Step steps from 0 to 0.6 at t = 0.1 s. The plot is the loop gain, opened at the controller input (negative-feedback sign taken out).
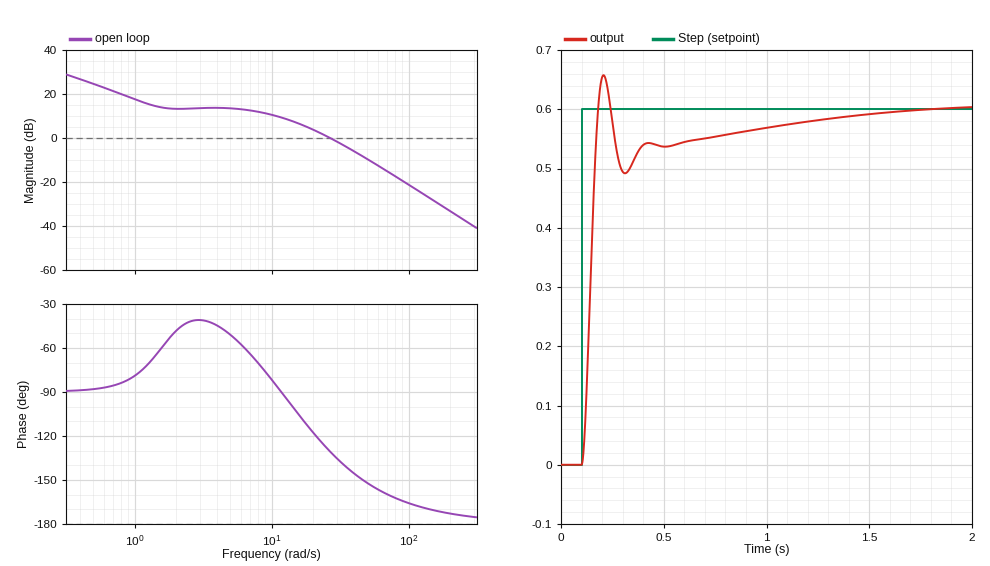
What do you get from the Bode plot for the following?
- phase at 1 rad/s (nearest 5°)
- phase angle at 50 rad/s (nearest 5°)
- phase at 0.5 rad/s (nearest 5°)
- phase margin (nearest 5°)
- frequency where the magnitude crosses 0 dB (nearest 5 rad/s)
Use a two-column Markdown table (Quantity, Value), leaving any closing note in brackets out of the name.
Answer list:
| Quantity | Value |
|---|---|
| phase at 1 rad/s | -80° |
| phase angle at 50 rad/s | -150° |
| phase at 0.5 rad/s | -90° |
| phase margin | 50° |
| frequency where the magnitude crosses 0 dB | 25 rad/s |
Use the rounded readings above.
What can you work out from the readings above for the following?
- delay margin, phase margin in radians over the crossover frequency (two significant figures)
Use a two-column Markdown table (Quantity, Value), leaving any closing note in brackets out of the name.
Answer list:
| Quantity | Value |
|---|---|
| delay margin, phase margin in radians over the crossover frequency | 0.035 s |
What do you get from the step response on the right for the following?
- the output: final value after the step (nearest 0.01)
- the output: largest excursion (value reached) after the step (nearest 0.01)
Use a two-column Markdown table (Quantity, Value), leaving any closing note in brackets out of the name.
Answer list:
| Quantity | Value |
|---|---|
| the output: final value after the step | 0.60 |
| the output: largest excursion (value reached) after the step | 0.66 |
